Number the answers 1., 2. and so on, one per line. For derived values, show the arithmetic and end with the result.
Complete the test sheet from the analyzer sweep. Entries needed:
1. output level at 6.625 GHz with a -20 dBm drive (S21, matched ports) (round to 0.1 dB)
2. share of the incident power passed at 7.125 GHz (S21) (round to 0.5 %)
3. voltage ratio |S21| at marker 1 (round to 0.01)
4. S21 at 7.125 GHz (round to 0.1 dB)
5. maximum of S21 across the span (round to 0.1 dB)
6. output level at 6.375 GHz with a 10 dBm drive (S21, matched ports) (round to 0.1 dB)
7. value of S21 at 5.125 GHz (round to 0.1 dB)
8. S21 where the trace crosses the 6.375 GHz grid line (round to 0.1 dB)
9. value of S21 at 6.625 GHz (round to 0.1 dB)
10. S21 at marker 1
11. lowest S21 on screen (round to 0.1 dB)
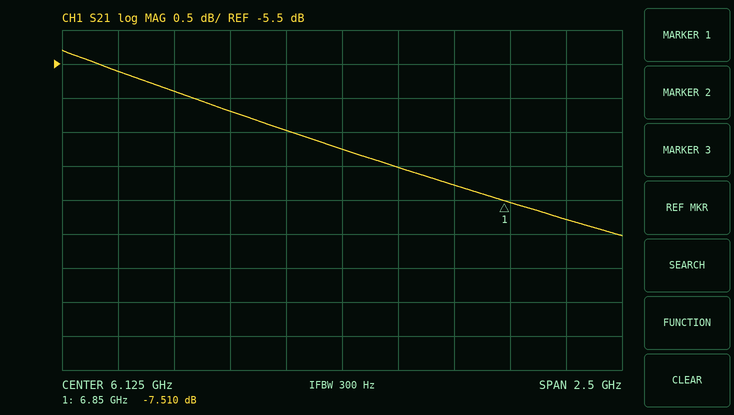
1. -20 dBm + (-7.3 dB) = -27.3 dBm
2. 10^(-7.8/10) ≈ 16.6 %, so 16.5 % to the nearest 0.5 %
3. 10^(-7.51/20) ≈ 0.42
4. -7.8 dB
5. -5.3 dB
6. 10 dBm + (-7.0 dB) = 3.0 dBm
7. -5.6 dB
8. -7.0 dB
9. -7.3 dB
10. -7.510 dB
11. -8.0 dB
